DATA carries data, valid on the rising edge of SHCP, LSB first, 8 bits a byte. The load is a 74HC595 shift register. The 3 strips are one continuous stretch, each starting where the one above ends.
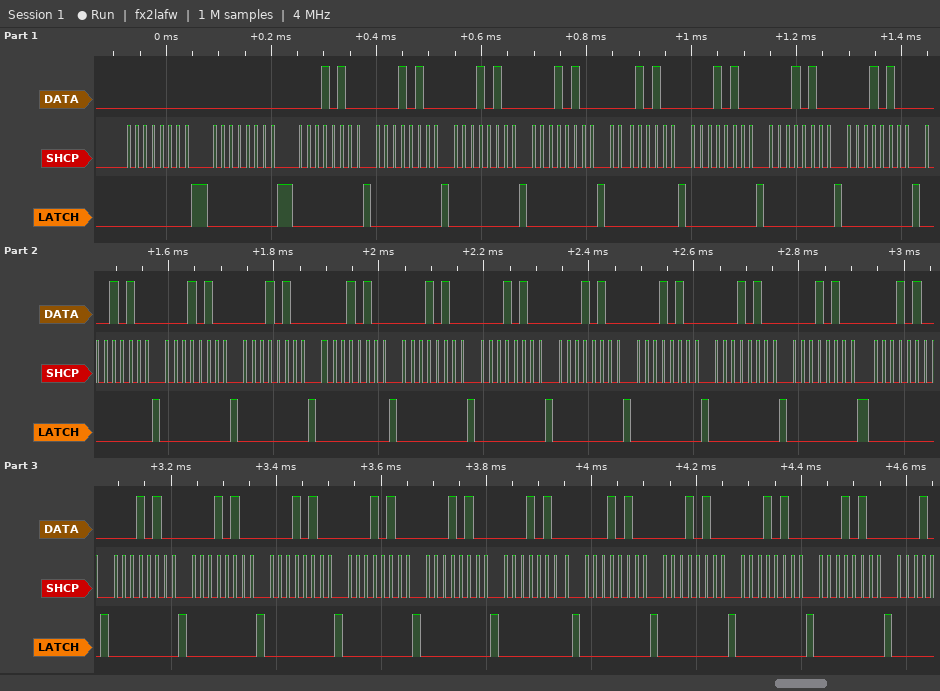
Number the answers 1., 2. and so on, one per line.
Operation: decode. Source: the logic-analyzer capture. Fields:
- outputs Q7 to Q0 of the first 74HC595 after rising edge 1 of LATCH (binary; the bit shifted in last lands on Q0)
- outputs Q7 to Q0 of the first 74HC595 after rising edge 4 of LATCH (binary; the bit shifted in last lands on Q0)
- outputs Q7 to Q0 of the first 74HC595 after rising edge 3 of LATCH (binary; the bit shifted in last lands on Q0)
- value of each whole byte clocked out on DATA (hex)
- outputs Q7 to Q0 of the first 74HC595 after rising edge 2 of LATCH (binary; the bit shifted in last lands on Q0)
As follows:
1. 00000000
2. 00010100
3. 00010100
4. 00 00 28 28 28 28 28 28 28 28 28 28 28 28 28 28 28 28 28 28 28 28 28 28 28 28 28 28 28 28 28
5. 00000000
